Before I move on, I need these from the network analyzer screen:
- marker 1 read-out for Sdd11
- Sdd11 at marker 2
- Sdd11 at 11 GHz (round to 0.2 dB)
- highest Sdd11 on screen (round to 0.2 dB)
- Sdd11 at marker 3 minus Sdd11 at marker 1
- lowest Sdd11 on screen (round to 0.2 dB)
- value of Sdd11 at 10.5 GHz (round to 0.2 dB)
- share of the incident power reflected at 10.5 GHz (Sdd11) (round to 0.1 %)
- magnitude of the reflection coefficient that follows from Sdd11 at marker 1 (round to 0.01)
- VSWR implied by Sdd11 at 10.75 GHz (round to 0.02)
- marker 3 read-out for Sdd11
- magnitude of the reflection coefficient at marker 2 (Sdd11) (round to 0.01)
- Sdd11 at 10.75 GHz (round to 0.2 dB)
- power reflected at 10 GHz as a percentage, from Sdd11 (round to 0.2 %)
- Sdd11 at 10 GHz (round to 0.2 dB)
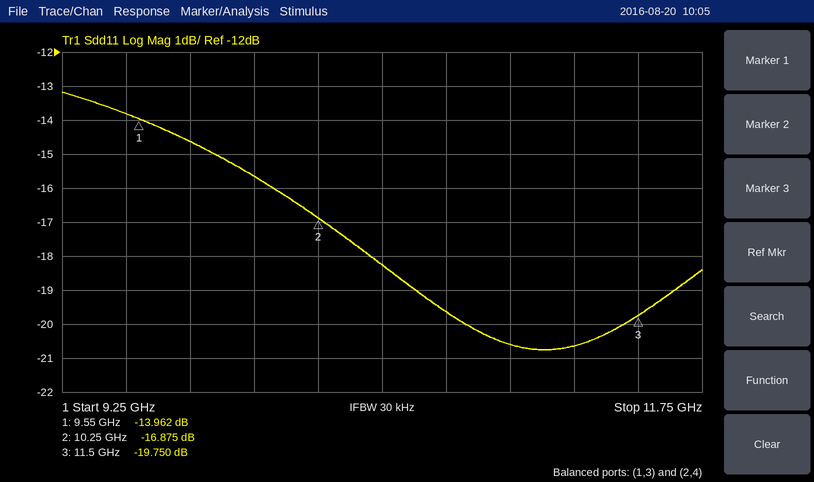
-13.962 dB
-16.875 dB
-20.6 dB
-13.2 dB
-5.788 dB
-20.8 dB
-18.2 dB
1.5 %
0.20
1.24
-19.750 dB
0.14
-19.6 dB
2.8 %
-15.6 dB
